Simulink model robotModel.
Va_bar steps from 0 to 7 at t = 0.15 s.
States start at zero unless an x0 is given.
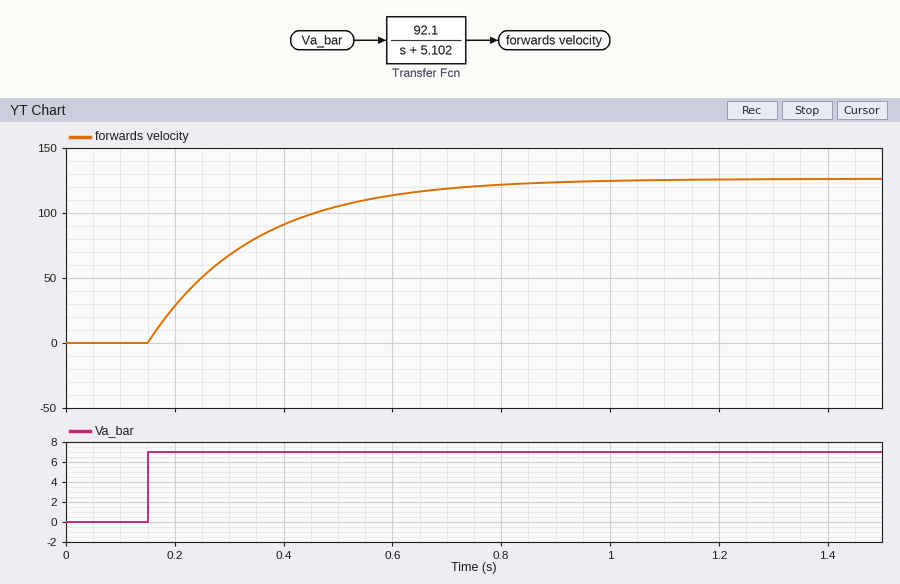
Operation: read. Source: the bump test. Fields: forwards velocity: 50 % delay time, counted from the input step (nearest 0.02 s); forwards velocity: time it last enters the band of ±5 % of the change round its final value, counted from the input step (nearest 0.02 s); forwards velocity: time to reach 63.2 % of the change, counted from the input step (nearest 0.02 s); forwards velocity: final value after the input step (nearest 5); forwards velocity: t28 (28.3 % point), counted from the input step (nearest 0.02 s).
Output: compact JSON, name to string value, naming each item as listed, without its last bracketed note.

{"forwards velocity: 50 % delay time, counted from the input step": "0.14 s", "forwards velocity: time it last enters the band of ±5 % of the change round its final value, counted from the input step": "0.58 s", "forwards velocity: time to reach 63.2 % of the change, counted from the input step": "0.20 s", "forwards velocity: final value after the input step": "125", "forwards velocity: t28 (28.3 % point), counted from the input step": "0.06 s"}
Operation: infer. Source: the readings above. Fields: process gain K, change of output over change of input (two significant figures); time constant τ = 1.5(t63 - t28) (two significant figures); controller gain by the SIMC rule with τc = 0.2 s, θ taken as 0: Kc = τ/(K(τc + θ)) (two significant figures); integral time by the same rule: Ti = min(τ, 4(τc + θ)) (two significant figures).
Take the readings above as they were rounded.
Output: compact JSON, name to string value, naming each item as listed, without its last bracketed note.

{"process gain K, change of output over change of input": "18", "time constant τ = 1.5(t63 - t28)": "0.21 s", "controller gain by the SIMC rule with τc = 0.2 s, θ taken as 0: Kc = τ/(K(τc + θ))": "0.058", "integral time by the same rule: Ti = min(τ, 4(τc + θ))": "0.21 s"}
